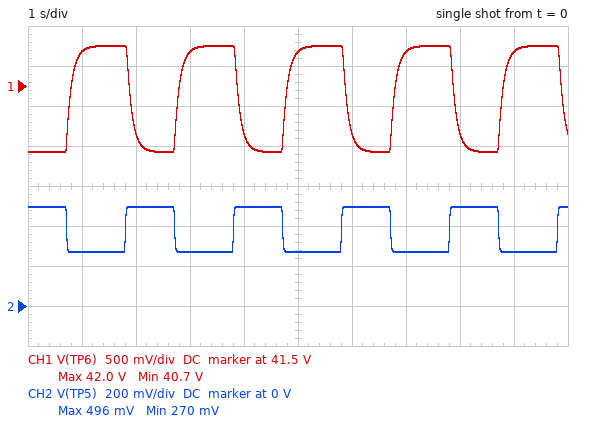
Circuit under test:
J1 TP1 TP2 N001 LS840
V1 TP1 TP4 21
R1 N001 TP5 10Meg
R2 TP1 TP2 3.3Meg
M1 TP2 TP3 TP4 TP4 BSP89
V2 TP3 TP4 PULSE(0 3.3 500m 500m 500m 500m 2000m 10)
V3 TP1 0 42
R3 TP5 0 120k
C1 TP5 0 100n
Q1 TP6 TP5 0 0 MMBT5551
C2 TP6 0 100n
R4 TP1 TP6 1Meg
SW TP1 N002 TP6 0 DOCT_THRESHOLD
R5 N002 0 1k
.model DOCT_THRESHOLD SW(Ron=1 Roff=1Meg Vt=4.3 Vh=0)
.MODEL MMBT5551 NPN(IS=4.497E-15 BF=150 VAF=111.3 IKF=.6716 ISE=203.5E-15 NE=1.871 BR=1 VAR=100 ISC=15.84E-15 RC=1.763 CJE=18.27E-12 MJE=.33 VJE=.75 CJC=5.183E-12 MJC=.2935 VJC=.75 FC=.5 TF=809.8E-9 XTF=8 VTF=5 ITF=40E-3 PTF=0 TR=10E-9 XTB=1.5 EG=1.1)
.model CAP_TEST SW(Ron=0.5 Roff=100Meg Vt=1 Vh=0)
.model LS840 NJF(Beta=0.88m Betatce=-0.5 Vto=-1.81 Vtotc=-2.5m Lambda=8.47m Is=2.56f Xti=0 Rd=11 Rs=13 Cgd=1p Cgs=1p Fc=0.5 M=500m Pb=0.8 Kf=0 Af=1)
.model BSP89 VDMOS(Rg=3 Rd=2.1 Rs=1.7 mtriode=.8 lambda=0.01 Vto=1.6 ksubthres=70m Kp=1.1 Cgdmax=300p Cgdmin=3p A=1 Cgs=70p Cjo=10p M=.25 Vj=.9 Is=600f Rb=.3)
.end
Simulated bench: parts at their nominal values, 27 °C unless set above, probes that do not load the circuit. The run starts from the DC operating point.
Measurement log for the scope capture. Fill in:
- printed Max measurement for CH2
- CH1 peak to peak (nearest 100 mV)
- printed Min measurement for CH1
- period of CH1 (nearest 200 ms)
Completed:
496 mV
1.3 V
40.7 V
2.0 s
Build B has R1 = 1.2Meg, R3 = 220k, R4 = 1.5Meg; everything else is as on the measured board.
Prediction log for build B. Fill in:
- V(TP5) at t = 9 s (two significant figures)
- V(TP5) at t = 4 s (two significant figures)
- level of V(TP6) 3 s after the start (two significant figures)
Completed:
600 mV
610 mV
35 mV
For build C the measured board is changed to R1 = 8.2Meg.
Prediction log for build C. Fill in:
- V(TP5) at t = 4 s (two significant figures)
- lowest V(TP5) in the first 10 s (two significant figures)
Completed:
580 mV
330 mV
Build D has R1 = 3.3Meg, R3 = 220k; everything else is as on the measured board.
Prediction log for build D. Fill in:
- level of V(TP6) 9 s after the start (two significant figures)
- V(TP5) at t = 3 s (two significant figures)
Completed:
68 mV
600 mV
